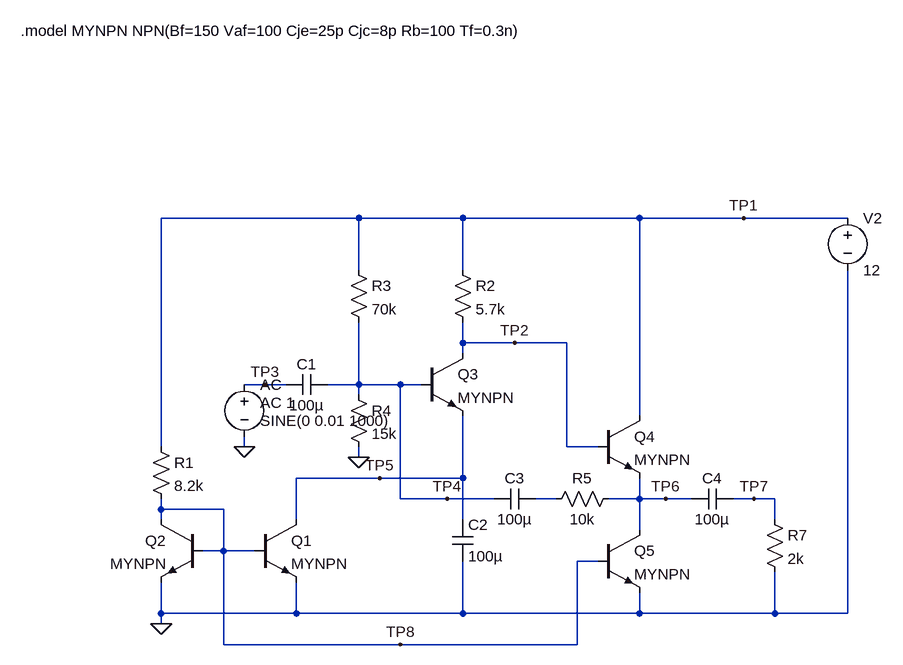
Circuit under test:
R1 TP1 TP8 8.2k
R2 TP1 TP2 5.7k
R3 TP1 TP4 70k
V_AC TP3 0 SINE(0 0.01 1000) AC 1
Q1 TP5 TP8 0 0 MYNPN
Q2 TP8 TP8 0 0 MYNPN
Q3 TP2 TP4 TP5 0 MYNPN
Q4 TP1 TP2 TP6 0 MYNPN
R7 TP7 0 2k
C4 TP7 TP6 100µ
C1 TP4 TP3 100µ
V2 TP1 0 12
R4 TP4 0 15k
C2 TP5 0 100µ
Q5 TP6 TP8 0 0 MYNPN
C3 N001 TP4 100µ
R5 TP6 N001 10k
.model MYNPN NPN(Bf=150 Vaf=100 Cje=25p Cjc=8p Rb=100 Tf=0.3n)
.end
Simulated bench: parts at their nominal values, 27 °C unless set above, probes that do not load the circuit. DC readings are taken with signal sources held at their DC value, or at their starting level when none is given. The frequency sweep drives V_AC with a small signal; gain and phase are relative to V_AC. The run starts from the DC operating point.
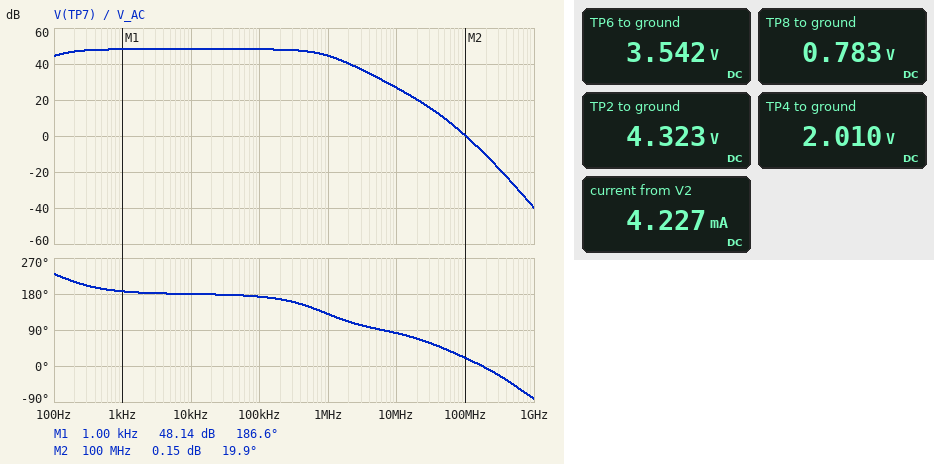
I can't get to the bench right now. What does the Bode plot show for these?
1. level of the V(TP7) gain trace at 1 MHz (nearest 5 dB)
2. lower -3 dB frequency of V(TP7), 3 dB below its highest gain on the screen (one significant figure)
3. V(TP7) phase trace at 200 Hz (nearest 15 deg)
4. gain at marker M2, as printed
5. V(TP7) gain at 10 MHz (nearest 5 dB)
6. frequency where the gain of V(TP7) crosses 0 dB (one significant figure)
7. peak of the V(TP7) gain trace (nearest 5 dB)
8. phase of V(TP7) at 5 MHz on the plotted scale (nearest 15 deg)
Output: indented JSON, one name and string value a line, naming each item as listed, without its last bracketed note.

{
  "level of the V(TP7) gain trace at 1 MHz": "45 dB",
  "lower -3 dB frequency of V(TP7), 3 dB below its highest gain on the screen": "100 Hz",
  "V(TP7) phase trace at 200 Hz": "210 deg",
  "gain at marker M2, as printed": "0.15 dB",
  "V(TP7) gain at 10 MHz": "25 dB",
  "frequency where the gain of V(TP7) crosses 0 dB": "100 MHz",
  "peak of the V(TP7) gain trace": "50 dB",
  "phase of V(TP7) at 5 MHz on the plotted scale": "90 deg"
}
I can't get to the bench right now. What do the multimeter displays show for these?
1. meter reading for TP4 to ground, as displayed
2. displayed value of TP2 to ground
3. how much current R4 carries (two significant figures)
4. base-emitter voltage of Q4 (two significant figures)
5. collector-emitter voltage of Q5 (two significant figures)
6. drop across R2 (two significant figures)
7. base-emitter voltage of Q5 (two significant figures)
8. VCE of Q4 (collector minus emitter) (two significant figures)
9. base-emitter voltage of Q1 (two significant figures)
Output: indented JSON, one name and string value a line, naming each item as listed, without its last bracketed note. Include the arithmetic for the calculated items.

{
  "meter reading for TP4 to ground, as displayed": "2.010 V",
  "displayed value of TP2 to ground": "4.323 V",
  "how much current R4 carries": "(2.01 V) / 15 kΩ = 130 µA",
  "base-emitter voltage of Q4": "4.323 V - 3.542 V = 780 mV",
  "collector-emitter voltage of Q5": "3.542 V = 3.5 V",
  "drop across R2": "12 V - 4.323 V = 7.7 V",
  "base-emitter voltage of Q5": "783 mV = 780 mV",
  "VCE of Q4 (collector minus emitter)": "12 V - 3.542 V = 8.5 V",
  "base-emitter voltage of Q1": "783 mV = 780 mV"
}
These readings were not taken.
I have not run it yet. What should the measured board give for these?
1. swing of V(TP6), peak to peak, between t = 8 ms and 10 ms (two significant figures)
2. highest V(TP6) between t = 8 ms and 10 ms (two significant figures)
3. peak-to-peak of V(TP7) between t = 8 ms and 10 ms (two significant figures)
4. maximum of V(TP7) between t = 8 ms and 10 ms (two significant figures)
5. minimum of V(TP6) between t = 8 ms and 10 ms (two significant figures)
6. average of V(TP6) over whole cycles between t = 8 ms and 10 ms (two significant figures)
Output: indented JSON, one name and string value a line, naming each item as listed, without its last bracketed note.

{
  "swing of V(TP6), peak to peak, between t = 8 ms and 10 ms": "4.6 V",
  "highest V(TP6) between t = 8 ms and 10 ms": "5.9 V",
  "peak-to-peak of V(TP7) between t = 8 ms and 10 ms": "4.6 V",
  "maximum of V(TP7) between t = 8 ms and 10 ms": "2.3 V",
  "minimum of V(TP6) between t = 8 ms and 10 ms": "1.3 V",
  "average of V(TP6) over whole cycles between t = 8 ms and 10 ms": "3.6 V"
}
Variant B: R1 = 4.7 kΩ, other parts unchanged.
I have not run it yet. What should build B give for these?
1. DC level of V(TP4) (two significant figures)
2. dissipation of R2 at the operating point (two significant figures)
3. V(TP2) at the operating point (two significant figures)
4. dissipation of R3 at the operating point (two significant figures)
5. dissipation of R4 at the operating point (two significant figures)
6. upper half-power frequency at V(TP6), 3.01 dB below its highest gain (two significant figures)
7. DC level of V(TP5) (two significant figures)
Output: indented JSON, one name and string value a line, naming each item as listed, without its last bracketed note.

{
  "DC level of V(TP4)": "1.4 V",
  "dissipation of R2 at the operating point": "22 mW",
  "V(TP2) at the operating point": "700 mV",
  "dissipation of R3 at the operating point": "1.6 mW",
  "dissipation of R4 at the operating point": "130 µW",
  "upper half-power frequency at V(TP6), 3.01 dB below its highest gain": "49 MHz",
  "DC level of V(TP5)": "600 mV"
}
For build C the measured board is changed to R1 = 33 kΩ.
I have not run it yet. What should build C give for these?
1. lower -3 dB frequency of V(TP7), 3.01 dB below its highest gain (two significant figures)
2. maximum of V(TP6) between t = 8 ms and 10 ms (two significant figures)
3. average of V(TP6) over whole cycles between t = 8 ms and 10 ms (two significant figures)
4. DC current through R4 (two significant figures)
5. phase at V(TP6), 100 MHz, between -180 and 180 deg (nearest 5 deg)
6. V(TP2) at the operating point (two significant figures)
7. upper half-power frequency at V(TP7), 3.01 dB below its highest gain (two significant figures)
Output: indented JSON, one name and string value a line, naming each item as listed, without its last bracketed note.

{
  "lower -3 dB frequency of V(TP7), 3.01 dB below its highest gain": "31 Hz",
  "maximum of V(TP6) between t = 8 ms and 10 ms": "9.9 V",
  "average of V(TP6) over whole cycles between t = 8 ms and 10 ms": "9.3 V",
  "DC current through R4": "140 µA",
  "phase at V(TP6), 100 MHz, between -180 and 180 deg": "10 deg",
  "V(TP2) at the operating point": "10 V",
  "upper half-power frequency at V(TP7), 3.01 dB below its highest gain": "1.9 MHz"
}
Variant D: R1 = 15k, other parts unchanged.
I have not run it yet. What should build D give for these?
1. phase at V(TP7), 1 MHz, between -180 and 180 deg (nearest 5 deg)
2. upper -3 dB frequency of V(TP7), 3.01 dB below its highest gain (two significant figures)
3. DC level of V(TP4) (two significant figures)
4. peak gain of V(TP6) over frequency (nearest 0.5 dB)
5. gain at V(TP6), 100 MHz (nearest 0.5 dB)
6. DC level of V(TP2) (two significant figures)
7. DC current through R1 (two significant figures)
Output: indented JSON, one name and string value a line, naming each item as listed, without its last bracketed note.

{
  "phase at V(TP7), 1 MHz, between -180 and 180 deg": "145 deg",
  "upper -3 dB frequency of V(TP7), 3.01 dB below its highest gain": "1.4 MHz",
  "DC level of V(TP4)": "2.1 V",
  "peak gain of V(TP6) over frequency": "43.5 dB",
  "gain at V(TP6), 100 MHz": "-2.0 dB",
  "DC level of V(TP2)": "7.8 V",
  "DC current through R1": "750 µA"
}
